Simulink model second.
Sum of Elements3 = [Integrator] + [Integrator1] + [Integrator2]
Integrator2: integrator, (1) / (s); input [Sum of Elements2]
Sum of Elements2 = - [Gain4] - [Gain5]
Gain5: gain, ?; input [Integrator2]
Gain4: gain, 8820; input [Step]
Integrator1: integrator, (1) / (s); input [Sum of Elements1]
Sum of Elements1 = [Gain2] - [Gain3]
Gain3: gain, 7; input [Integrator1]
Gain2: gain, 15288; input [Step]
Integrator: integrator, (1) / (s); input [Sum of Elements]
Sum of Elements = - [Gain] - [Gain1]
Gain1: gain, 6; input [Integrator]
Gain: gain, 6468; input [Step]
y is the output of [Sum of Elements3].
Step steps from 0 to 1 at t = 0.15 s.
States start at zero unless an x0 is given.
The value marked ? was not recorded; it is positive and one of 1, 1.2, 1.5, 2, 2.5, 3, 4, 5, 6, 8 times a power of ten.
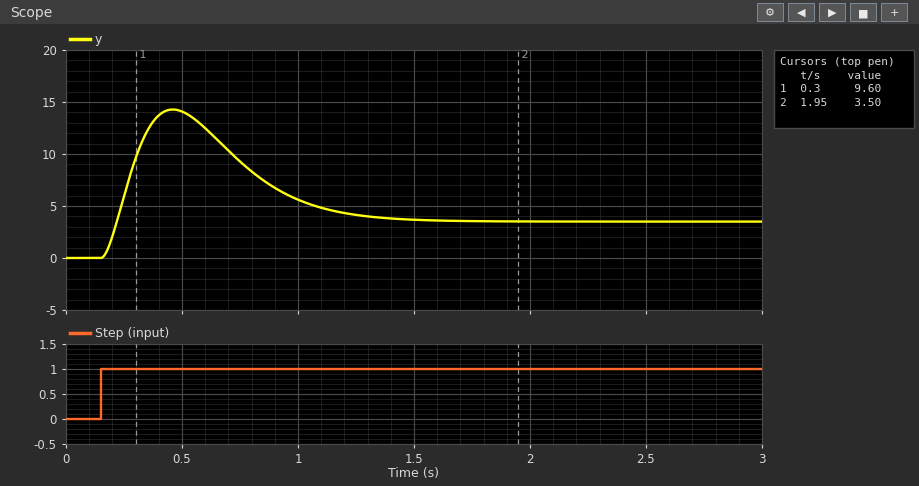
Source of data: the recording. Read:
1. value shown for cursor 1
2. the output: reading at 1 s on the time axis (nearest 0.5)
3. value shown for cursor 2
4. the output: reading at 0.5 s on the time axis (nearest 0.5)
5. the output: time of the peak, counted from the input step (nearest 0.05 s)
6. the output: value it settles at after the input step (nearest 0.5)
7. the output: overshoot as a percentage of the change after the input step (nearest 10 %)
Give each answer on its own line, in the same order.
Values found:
9.60
5.5
3.50
14.0
0.30 s
3.5
310 %
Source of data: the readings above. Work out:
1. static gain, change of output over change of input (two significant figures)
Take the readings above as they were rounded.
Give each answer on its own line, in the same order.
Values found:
3.5
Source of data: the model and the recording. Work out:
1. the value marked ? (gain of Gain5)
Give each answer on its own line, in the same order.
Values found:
8
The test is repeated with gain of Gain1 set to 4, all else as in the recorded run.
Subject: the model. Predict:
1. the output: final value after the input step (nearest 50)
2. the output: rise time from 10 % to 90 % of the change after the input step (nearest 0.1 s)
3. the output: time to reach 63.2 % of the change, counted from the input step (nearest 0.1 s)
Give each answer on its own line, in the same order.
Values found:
-550
0.7 s
0.5 s
